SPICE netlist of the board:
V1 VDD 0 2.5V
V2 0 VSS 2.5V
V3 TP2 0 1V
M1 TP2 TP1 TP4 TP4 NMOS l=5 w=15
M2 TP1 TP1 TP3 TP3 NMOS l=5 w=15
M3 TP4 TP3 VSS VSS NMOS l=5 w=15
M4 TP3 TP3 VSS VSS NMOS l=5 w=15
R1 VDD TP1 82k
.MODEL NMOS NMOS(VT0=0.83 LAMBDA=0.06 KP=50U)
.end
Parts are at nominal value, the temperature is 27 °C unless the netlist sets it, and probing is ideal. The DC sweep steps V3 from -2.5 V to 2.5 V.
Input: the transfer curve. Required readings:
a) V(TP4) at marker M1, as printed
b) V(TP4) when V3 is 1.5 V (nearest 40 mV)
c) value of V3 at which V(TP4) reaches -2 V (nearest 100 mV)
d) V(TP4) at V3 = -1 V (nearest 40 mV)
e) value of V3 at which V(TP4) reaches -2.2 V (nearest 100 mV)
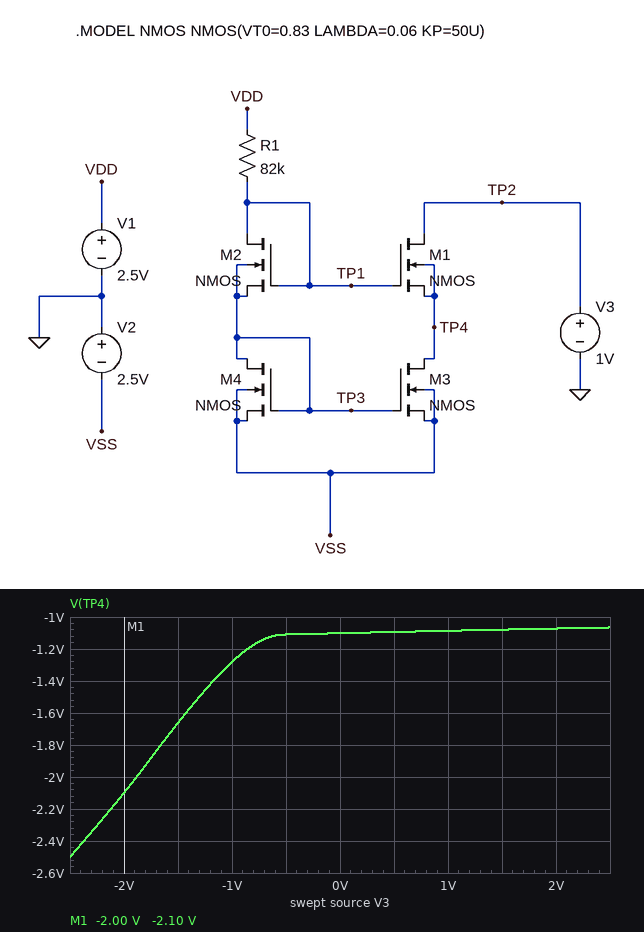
-2.10 V
-1.08 V
-1.9 V
-1.28 V
-2.1 V
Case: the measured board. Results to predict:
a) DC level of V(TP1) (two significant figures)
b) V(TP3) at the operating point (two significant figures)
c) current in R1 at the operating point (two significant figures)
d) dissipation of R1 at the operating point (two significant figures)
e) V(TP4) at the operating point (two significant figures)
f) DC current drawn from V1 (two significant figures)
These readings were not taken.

310 mV
-1.1 V
27 µA
59 µW
-1.1 V
27 µA
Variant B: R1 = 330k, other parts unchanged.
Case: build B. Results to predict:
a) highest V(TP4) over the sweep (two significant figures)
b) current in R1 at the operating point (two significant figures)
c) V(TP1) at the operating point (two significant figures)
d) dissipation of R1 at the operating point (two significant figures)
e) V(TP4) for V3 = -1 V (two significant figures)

-1.3 V
8.2 µA
-200 mV
22 µW
-1.4 V
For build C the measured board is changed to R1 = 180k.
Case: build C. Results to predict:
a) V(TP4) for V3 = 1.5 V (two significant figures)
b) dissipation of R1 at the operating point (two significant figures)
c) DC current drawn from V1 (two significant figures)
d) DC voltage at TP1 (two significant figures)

-1.2 V
35 µW
14 µA
-8.4 mV
